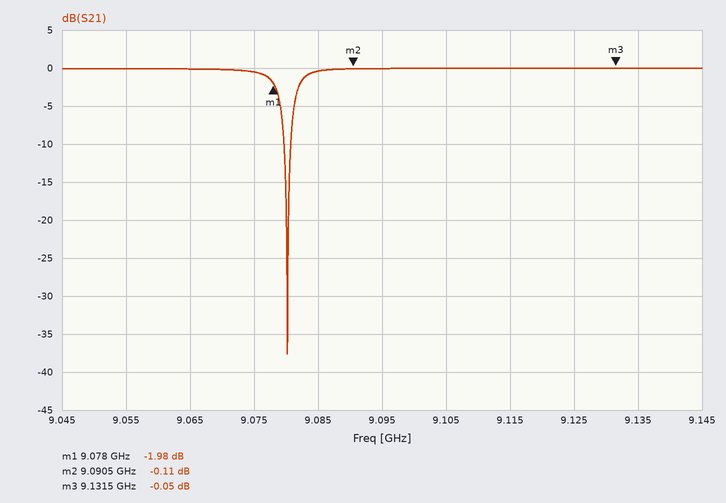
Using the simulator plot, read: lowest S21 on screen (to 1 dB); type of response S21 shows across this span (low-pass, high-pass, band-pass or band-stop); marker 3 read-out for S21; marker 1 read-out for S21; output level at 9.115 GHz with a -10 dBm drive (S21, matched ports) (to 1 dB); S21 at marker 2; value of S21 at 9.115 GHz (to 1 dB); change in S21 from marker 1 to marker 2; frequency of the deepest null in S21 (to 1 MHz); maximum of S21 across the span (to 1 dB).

-38 dB
band-stop
-0.05 dB
-1.98 dB
-10 dBm
-0.11 dB
0 dB
1.87 dB
9.080 GHz
0 dB
